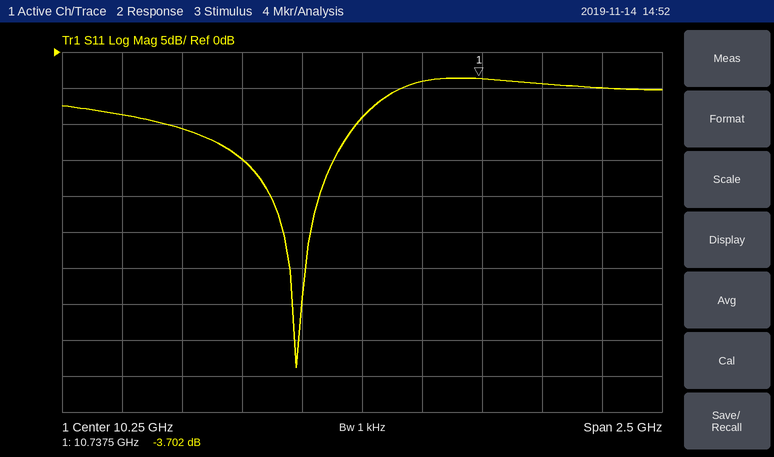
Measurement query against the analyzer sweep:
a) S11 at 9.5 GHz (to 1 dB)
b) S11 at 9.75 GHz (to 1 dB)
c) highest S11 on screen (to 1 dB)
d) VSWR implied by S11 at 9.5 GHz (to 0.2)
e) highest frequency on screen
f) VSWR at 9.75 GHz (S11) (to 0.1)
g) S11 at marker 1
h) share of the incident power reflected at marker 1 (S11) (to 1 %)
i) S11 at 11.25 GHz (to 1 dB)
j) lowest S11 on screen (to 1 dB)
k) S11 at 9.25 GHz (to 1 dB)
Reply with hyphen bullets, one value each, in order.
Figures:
- -11 dB
- -15 dB
- -4 dB
- 1.8
- 11.5 GHz
- 1.4
- -3.702 dB
- 43 %
- -5 dB
- -44 dB
- -9 dB
